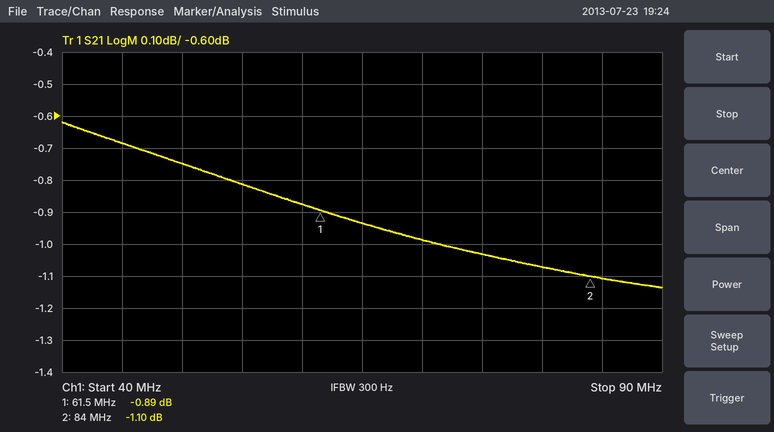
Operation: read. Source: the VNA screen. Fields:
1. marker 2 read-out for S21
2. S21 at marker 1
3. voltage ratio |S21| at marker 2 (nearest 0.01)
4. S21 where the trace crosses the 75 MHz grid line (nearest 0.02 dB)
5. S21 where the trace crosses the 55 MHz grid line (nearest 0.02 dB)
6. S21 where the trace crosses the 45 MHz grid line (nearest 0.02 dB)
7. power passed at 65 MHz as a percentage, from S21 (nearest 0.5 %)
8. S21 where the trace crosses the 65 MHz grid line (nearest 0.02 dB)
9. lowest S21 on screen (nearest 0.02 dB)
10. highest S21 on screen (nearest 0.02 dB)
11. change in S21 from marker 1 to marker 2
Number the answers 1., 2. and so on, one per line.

1. -1.10 dB
2. -0.89 dB
3. 0.88
4. -1.04 dB
5. -0.82 dB
6. -0.68 dB
7. 80.5 %
8. -0.94 dB
9. -1.14 dB
10. -0.62 dB
11. -0.21 dB
